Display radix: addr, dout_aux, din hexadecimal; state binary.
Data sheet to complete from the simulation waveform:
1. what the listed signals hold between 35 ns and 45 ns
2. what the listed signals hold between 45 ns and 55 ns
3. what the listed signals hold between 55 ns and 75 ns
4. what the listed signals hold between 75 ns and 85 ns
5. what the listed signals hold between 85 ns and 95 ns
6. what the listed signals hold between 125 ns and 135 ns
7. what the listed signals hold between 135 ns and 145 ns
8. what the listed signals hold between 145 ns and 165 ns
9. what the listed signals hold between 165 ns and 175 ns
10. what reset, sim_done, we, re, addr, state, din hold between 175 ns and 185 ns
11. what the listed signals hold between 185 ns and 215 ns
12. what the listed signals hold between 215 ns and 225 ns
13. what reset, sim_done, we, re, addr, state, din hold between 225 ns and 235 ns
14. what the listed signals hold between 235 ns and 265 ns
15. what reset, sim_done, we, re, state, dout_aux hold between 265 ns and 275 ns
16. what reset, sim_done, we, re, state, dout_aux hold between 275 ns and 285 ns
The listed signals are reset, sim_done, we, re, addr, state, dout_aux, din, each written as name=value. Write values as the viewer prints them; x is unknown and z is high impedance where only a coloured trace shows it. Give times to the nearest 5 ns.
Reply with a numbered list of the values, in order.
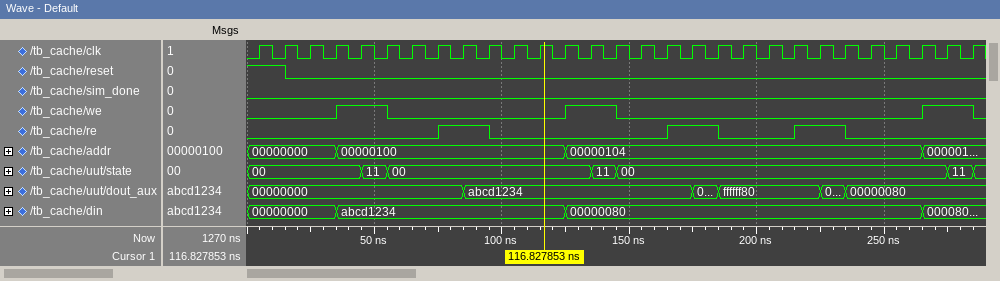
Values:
1. reset=0, sim_done=0, we=1, re=0, addr=00000100, state=00, dout_aux=00000000, din=abcd1234
2. reset=0, sim_done=0, we=1, re=0, addr=00000100, state=11, dout_aux=00000000, din=abcd1234
3. reset=0, sim_done=0, we=0, re=0, addr=00000100, state=00, dout_aux=00000000, din=abcd1234
4. reset=0, sim_done=0, we=0, re=1, addr=00000100, state=00, dout_aux=00000000, din=abcd1234
5. reset=0, sim_done=0, we=0, re=1, addr=00000100, state=00, dout_aux=abcd1234, din=abcd1234
6. reset=0, sim_done=0, we=1, re=0, addr=00000104, state=00, dout_aux=abcd1234, din=00000080
7. reset=0, sim_done=0, we=1, re=0, addr=00000104, state=11, dout_aux=abcd1234, din=00000080
8. reset=0, sim_done=0, we=0, re=0, addr=00000104, state=00, dout_aux=abcd1234, din=00000080
9. reset=0, sim_done=0, we=0, re=1, addr=00000104, state=00, dout_aux=abcd1234, din=00000080
10. reset=0, sim_done=0, we=0, re=1, addr=00000104, state=00, din=00000080
11. reset=0, sim_done=0, we=0, re=0, addr=00000104, state=00, dout_aux=ffffff80, din=00000080
12. reset=0, sim_done=0, we=0, re=1, addr=00000104, state=00, dout_aux=ffffff80, din=00000080
13. reset=0, sim_done=0, we=0, re=1, addr=00000104, state=00, din=00000080
14. reset=0, sim_done=0, we=0, re=0, addr=00000104, state=00, dout_aux=00000080, din=00000080
15. reset=0, sim_done=0, we=1, re=0, state=00, dout_aux=00000080
16. reset=0, sim_done=0, we=1, re=0, state=11, dout_aux=00000080
